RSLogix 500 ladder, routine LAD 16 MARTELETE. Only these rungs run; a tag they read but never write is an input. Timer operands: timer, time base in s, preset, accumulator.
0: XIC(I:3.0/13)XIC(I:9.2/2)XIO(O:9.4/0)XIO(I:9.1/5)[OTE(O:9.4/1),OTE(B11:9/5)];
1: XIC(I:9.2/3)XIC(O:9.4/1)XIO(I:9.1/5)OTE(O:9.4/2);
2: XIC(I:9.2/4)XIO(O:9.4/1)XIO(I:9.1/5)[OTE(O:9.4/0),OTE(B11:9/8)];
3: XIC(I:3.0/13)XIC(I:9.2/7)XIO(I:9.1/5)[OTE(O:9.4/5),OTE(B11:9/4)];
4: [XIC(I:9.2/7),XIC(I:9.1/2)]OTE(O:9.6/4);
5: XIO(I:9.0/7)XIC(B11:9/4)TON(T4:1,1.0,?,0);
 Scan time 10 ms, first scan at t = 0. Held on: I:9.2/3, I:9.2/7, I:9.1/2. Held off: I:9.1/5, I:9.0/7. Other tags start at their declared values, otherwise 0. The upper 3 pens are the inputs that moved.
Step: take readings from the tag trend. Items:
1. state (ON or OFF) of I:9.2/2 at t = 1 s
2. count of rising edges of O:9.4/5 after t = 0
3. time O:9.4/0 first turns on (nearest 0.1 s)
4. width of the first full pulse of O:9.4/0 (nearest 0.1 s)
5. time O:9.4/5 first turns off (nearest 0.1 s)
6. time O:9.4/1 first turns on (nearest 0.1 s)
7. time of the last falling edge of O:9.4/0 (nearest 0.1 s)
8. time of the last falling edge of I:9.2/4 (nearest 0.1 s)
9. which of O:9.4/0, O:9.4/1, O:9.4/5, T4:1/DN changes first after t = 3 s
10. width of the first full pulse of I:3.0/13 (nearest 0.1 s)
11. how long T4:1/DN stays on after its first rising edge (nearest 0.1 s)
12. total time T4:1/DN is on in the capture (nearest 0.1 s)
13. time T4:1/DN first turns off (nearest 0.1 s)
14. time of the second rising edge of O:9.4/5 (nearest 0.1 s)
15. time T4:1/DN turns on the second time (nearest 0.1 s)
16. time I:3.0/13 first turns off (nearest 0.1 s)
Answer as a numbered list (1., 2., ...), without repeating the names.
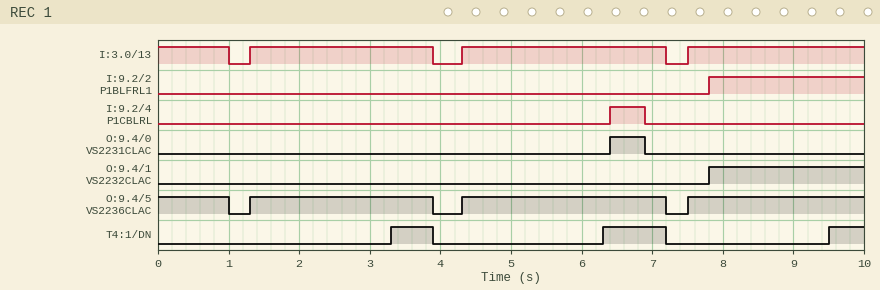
1. OFF
2. 3
3. 6.4 s
4. 0.5 s
5. 1.0 s
6. 7.8 s
7. 6.9 s
8. 6.9 s
9. T4:1/DN
10. 2.6 s
11. 0.6 s
12. 2.0 s
13. 3.9 s
14. 4.3 s
15. 6.3 s
16. 1.0 s
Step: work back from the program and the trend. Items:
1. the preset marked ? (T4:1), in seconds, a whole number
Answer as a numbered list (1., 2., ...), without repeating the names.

1. 2 s
